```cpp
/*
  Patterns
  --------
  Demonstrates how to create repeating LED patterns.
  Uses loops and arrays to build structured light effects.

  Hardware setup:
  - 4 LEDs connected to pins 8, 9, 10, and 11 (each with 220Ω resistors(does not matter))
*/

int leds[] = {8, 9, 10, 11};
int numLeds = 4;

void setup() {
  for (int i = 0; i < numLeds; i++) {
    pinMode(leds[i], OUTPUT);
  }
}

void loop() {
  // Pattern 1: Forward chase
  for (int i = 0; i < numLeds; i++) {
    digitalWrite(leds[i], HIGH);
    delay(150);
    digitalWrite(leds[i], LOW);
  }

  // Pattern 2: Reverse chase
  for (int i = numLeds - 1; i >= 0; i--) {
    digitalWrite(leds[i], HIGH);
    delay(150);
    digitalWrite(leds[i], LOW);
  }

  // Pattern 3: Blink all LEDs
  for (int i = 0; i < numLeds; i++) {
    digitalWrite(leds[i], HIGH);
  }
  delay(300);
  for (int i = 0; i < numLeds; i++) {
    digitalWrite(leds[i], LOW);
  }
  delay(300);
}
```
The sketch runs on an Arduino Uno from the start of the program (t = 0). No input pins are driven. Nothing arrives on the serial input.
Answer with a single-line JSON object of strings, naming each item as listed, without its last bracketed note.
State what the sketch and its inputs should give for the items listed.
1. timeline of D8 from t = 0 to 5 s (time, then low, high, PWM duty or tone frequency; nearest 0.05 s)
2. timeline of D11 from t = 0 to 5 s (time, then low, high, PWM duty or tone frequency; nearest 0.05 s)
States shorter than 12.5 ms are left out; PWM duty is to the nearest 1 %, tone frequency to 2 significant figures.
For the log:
{"timeline of D8 from t = 0 to 5 s": "0 s high; 0.15 s low; 1.05 s high; 1.5 s low; 1.8 s high; 1.95 s low; 2.85 s high; 3.3 s low; 3.6 s high; 3.75 s low; 4.65 s high", "timeline of D11 from t = 0 to 5 s": "0 s low; 0.45 s high; 0.75 s low; 1.2 s high; 1.5 s low; 2.25 s high; 2.55 s low; 3 s high; 3.3 s low; 4.05 s high; 4.35 s low; 4.8 s high"}
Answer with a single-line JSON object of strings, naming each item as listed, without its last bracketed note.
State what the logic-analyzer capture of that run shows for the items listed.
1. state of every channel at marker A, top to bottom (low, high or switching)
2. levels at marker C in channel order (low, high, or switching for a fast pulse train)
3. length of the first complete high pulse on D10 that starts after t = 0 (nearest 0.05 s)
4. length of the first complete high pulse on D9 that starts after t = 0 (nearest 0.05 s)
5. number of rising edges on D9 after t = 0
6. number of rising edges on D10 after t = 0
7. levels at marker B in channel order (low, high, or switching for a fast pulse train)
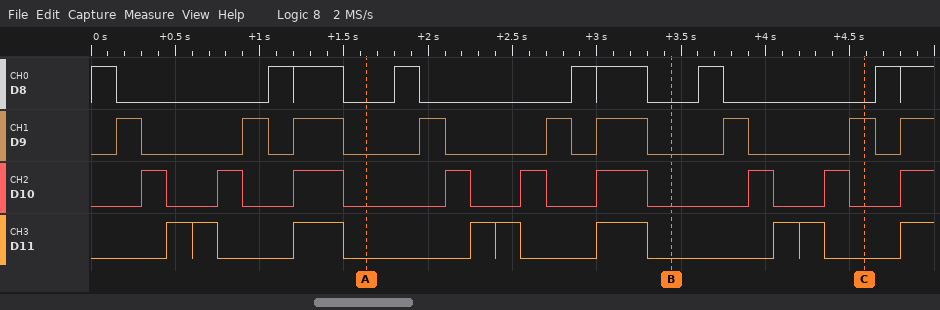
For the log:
{"state of every channel at marker A, top to bottom": "D8 low, D9 low, D10 low, D11 low", "levels at marker C in channel order": "D8 low, D9 high, D10 low, D11 low", "length of the first complete high pulse on D10 that starts after t = 0": "0.15 s", "length of the first complete high pulse on D9 that starts after t = 0": "0.15 s", "number of rising edges on D9 after t = 0": "9", "number of rising edges on D10 after t = 0": "9", "levels at marker B in channel order": "D8 low, D9 low, D10 low, D11 low"}
